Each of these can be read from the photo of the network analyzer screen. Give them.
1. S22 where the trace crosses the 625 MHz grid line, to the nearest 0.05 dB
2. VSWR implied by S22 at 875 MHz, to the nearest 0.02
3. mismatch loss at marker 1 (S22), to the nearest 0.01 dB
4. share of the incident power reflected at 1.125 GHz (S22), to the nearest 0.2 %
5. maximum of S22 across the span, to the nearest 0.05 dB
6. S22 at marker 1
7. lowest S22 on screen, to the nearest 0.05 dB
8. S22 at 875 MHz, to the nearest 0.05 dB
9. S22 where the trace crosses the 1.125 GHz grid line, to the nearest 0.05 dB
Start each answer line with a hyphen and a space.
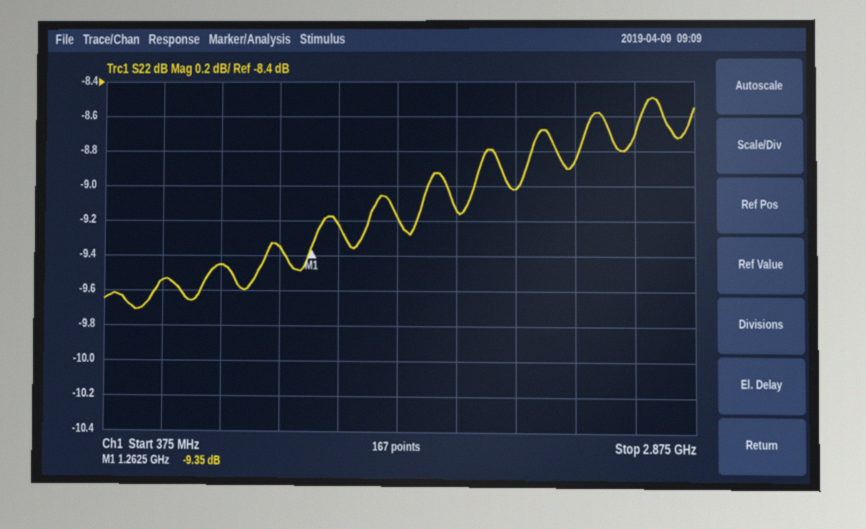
- -9.55 dB
- 2.02
- 0.54 dB
- 11.6 %
- -8.50 dB
- -9.35 dB
- -9.70 dB
- -9.45 dB
- -9.35 dB
